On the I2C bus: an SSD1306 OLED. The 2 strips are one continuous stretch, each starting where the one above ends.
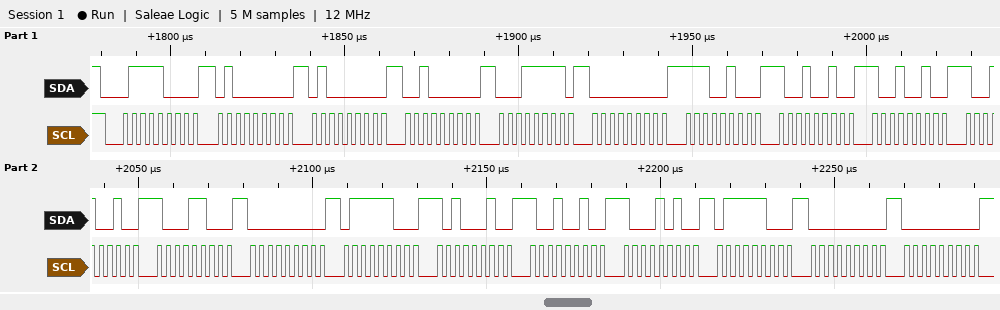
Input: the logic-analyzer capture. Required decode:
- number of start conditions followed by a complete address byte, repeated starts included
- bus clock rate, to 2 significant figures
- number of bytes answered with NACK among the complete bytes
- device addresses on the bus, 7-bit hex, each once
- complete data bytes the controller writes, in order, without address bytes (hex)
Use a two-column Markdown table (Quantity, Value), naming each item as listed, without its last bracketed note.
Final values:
| Quantity | Value |
|---|---|
| number of start conditions followed by a complete address byte, repeated starts included | 1 |
| bus clock rate, to 2 significant figures | 400 kHz |
| number of bytes answered with NACK among the complete bytes | 0 |
| device addresses on the bus, 7-bit hex, each once | 0x3C |
| complete data bytes the controller writes, in order, without address bytes | 40 40 20 1F 00 E4 92 92 92 8C 00 7C A2 92 8A 7C 00 00 |
